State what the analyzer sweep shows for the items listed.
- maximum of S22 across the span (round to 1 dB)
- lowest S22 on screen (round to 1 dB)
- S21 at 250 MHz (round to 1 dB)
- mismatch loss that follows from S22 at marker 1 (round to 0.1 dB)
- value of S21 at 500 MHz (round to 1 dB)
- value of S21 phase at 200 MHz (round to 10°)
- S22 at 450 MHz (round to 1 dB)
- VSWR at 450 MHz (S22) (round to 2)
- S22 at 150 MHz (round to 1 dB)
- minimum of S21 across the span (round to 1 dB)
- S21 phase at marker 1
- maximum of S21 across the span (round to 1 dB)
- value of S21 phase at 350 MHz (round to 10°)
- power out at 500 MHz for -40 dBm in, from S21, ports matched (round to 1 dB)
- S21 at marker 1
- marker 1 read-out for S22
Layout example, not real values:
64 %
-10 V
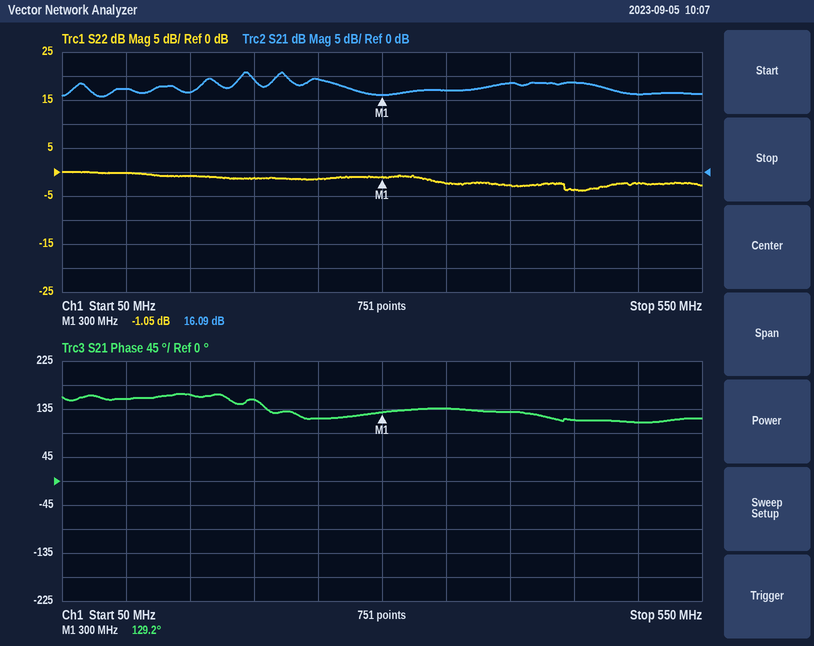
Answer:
0 dB
-4 dB
19 dB
6.7 dB
16 dB
150°
-4 dB
4
-1 dB
16 dB
129.2°
21 dB
140°
-24 dBm
16.09 dB
-1.05 dB
